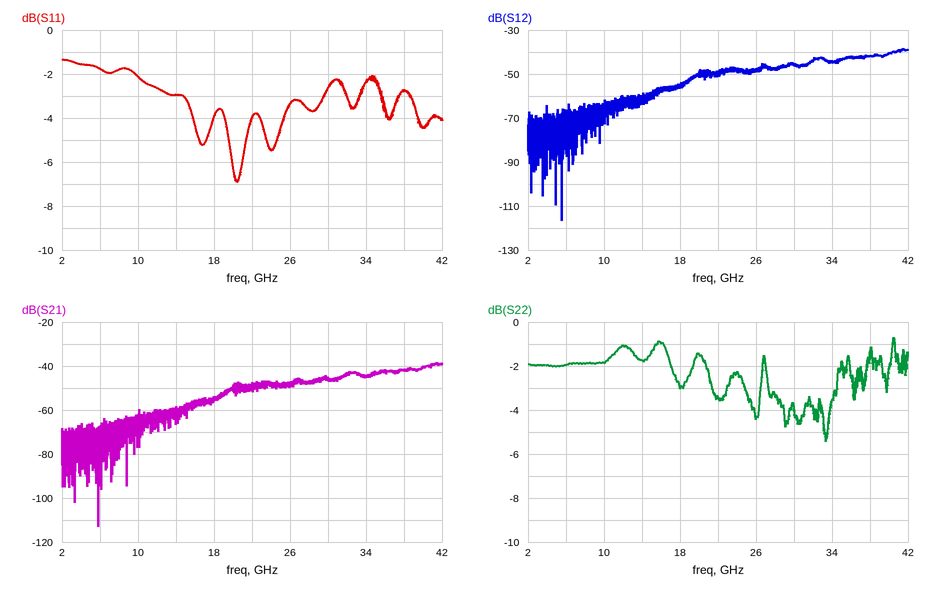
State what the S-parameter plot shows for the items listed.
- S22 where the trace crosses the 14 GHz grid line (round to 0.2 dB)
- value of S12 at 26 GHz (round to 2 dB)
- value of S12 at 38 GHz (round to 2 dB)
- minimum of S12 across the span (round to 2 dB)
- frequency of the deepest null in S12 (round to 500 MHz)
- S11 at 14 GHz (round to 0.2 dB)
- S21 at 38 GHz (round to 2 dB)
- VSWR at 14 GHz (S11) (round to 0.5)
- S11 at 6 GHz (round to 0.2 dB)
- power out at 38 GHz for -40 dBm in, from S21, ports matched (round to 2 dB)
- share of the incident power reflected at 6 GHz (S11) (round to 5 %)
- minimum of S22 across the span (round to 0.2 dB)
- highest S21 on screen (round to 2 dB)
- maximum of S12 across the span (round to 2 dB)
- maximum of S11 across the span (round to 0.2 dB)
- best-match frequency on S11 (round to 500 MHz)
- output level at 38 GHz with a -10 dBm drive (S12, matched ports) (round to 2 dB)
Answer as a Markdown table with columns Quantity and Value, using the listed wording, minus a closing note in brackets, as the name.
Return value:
| Quantity | Value |
|---|---|
| S22 where the trace crosses the 14 GHz grid line | -1.8 dB |
| value of S12 at 26 GHz | -48 dB |
| value of S12 at 38 GHz | -42 dB |
| minimum of S12 across the span | -116 dB |
| frequency of the deepest null in S12 | 5.5 GHz |
| S11 at 14 GHz | -3.0 dB |
| S21 at 38 GHz | -42 dB |
| VSWR at 14 GHz (S11) | 6.0 |
| S11 at 6 GHz | -1.8 dB |
| power out at 38 GHz for -40 dBm in, from S21, ports matched | -82 dBm |
| share of the incident power reflected at 6 GHz (S11) | 65 % |
| minimum of S22 across the span | -5.4 dB |
| highest S21 on screen | -38 dB |
| maximum of S12 across the span | -38 dB |
| maximum of S11 across the span | -1.4 dB |
| best-match frequency on S11 | 20.5 GHz |
| output level at 38 GHz with a -10 dBm drive (S12, matched ports) | -52 dBm |
